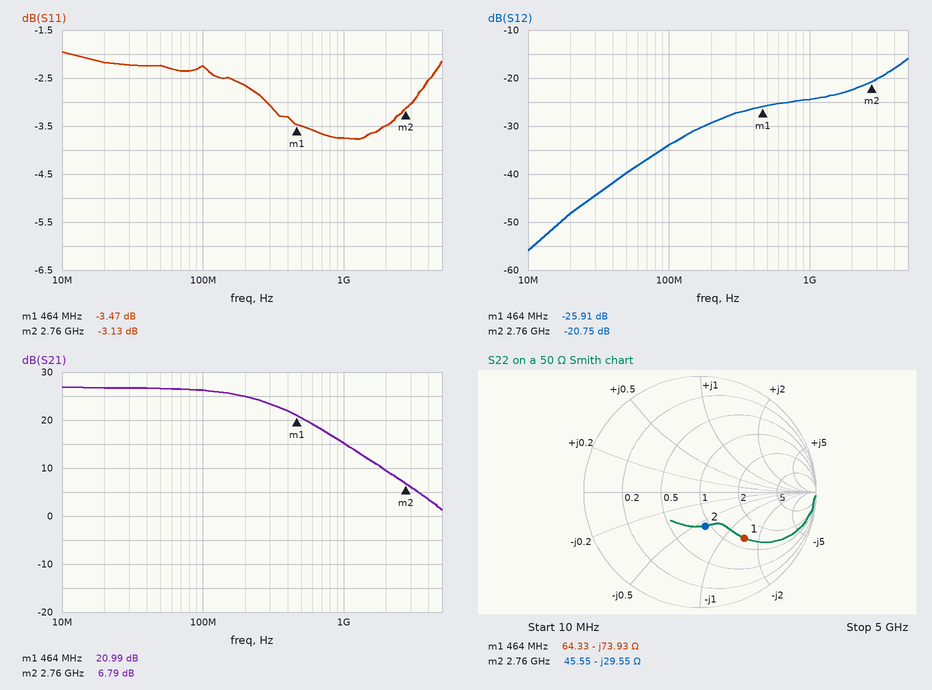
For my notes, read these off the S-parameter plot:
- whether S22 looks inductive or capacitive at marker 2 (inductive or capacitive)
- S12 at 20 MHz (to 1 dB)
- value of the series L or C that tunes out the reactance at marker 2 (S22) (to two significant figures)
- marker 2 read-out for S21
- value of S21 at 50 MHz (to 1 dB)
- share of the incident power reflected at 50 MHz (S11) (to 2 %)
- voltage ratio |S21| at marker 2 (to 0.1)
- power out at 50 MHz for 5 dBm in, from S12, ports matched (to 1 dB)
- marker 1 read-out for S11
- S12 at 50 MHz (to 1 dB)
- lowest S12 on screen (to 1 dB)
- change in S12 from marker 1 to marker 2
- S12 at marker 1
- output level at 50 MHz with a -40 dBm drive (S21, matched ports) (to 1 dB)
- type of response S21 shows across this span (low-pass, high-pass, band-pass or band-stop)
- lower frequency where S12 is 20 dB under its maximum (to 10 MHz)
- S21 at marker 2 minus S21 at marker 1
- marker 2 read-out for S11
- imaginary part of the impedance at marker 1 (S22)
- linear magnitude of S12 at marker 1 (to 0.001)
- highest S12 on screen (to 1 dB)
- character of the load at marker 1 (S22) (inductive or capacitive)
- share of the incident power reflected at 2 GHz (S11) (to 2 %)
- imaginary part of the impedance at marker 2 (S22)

capacitive
-48 dB
1.7 nH
6.79 dB
27 dB
60 %
2.2
-35 dBm
-3.47 dB
-40 dB
-56 dB
5.16 dB
-25.91 dB
-13 dBm
low-pass
80 MHz
-14.20 dB
-3.13 dB
-73.93 Ω
0.051
-16 dB
capacitive
44 %
-29.55 Ω
